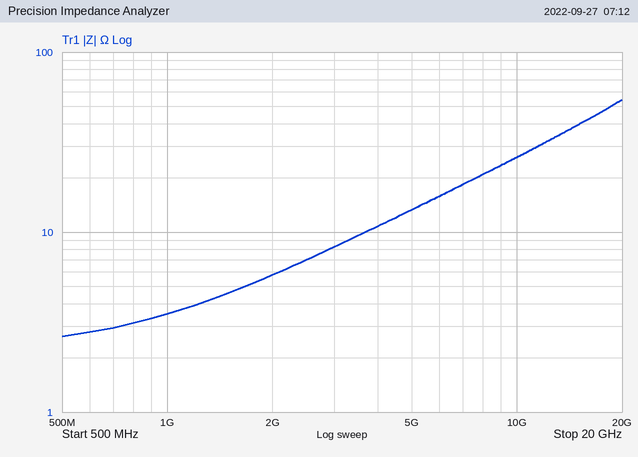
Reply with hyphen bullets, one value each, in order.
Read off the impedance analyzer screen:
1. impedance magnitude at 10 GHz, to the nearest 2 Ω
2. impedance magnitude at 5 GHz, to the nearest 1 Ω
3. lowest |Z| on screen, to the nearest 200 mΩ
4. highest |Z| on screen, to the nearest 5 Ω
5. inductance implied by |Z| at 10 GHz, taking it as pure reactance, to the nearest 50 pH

- 26 Ω
- 13 Ω
- 2.6 Ω
- 55 Ω
- 400 pH
